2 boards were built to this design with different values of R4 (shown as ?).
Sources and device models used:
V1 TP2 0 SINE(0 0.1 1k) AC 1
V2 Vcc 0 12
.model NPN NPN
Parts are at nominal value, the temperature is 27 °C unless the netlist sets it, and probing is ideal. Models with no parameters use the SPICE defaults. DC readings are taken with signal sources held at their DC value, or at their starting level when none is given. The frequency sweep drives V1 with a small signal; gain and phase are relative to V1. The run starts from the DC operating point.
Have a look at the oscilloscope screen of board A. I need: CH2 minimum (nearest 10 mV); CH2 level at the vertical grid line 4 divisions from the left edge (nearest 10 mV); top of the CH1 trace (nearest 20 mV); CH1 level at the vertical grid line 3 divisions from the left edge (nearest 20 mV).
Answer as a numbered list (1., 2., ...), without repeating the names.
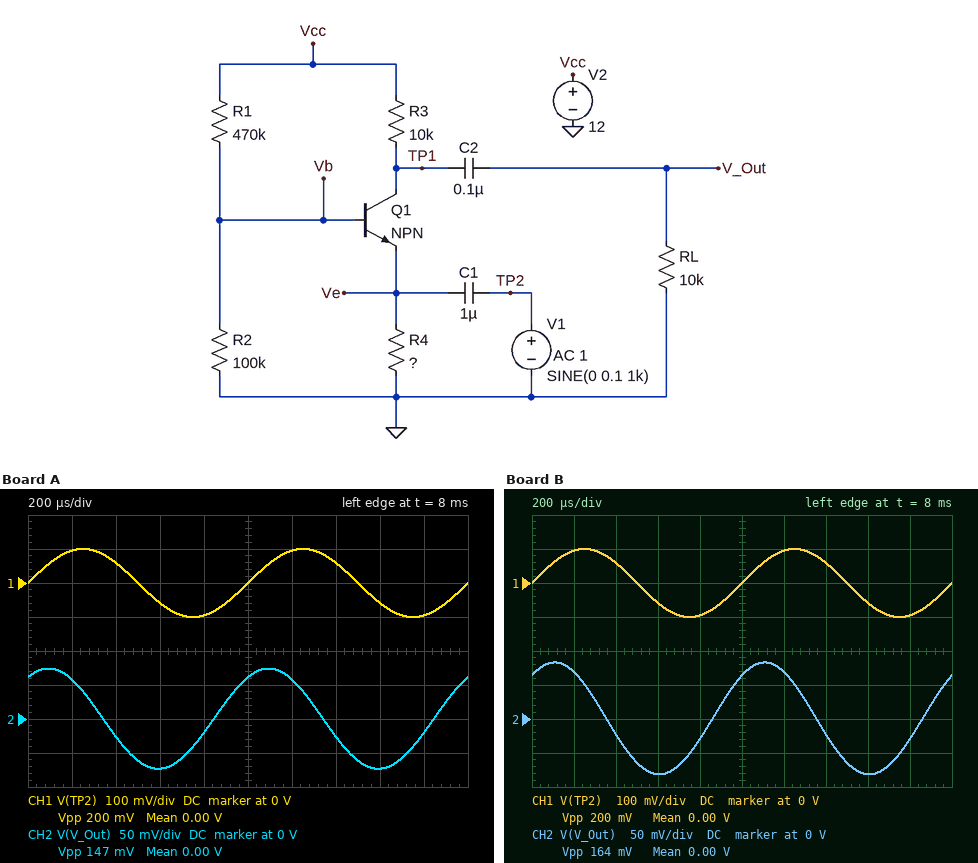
1. -70 mV
2. -20 mV
3. 100 mV
4. -60 mV
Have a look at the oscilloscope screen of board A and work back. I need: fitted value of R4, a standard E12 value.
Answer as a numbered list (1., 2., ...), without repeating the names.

1. 150 Ω
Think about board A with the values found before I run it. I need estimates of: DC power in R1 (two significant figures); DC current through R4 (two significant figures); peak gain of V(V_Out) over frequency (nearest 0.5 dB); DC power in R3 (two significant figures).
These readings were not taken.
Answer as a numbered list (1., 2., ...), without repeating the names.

1. 260 µW
2. 1.2 mA
3. 1.0 dB
4. 14 mW
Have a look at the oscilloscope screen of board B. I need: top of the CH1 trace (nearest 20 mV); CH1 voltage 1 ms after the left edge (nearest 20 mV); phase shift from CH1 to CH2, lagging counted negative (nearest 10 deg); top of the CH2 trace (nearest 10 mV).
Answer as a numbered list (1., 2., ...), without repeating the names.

1. 100 mV
2. 0 V
3. 50 deg
4. 80 mV
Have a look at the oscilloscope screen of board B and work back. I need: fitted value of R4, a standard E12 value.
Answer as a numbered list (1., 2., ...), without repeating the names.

1. 180 Ω
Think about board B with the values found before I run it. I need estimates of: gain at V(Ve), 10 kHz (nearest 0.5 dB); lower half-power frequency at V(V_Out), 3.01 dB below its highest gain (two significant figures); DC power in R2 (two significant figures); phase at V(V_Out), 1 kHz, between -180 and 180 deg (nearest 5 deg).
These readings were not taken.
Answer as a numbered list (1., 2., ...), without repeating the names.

1. 0 dB
2. 950 Hz
3. 9.8 µW
4. 50 deg
